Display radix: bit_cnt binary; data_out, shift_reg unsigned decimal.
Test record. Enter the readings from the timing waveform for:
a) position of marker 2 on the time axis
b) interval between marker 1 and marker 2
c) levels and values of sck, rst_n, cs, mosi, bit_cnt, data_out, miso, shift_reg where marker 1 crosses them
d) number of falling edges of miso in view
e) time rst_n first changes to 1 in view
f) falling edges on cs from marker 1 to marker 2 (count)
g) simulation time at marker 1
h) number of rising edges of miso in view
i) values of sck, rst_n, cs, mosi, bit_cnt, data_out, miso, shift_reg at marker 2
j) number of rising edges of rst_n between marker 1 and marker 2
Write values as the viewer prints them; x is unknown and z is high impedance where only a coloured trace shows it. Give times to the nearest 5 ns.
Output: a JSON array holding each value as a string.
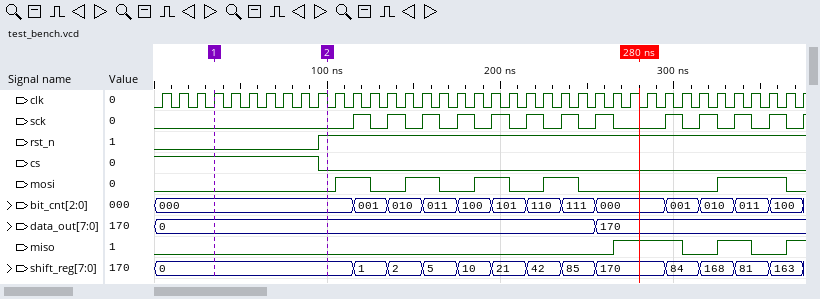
["100 ns", "65 ns", "sck=0, rst_n=0, cs=1, mosi=0, bit_cnt=000, data_out=0, miso=0, shift_reg=0", "2", "95 ns", "1", "35 ns", "3", "sck=0, rst_n=1, cs=0, mosi=0, bit_cnt=000, data_out=0, miso=0, shift_reg=0", "1"]
